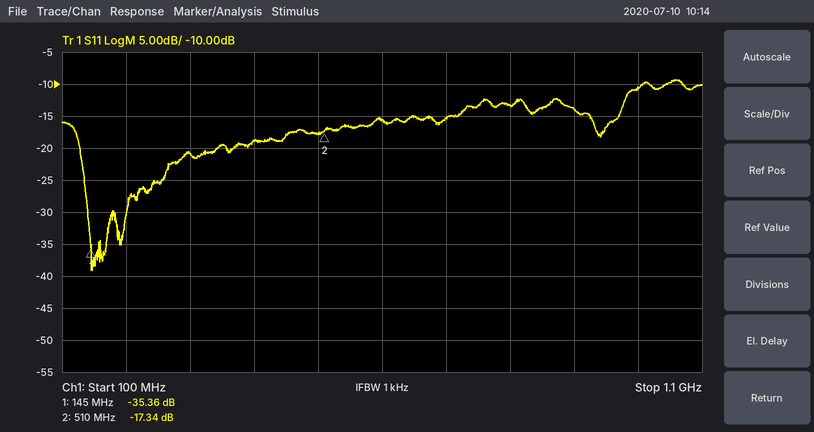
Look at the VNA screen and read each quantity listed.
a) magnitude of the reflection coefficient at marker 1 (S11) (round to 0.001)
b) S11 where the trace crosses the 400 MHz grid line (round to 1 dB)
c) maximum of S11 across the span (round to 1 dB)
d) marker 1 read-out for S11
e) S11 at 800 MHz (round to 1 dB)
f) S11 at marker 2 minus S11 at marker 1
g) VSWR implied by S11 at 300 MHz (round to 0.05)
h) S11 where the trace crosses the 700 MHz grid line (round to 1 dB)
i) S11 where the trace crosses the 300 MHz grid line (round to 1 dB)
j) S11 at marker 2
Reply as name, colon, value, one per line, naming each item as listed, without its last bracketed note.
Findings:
magnitude of the reflection coefficient at marker 1 (S11): 0.017
S11 where the trace crosses the 400 MHz grid line: -19 dB
maximum of S11 across the span: -9 dB
marker 1 read-out for S11: -35.36 dB
S11 at 800 MHz: -13 dB
S11 at marker 2 minus S11 at marker 1: 18.02 dB
VSWR implied by S11 at 300 MHz: 1.20
S11 where the trace crosses the 700 MHz grid line: -15 dB
S11 where the trace crosses the 300 MHz grid line: -21 dB
S11 at marker 2: -17.34 dB
